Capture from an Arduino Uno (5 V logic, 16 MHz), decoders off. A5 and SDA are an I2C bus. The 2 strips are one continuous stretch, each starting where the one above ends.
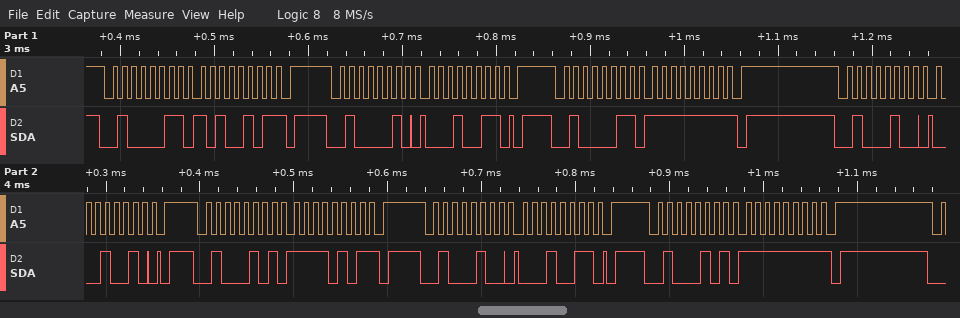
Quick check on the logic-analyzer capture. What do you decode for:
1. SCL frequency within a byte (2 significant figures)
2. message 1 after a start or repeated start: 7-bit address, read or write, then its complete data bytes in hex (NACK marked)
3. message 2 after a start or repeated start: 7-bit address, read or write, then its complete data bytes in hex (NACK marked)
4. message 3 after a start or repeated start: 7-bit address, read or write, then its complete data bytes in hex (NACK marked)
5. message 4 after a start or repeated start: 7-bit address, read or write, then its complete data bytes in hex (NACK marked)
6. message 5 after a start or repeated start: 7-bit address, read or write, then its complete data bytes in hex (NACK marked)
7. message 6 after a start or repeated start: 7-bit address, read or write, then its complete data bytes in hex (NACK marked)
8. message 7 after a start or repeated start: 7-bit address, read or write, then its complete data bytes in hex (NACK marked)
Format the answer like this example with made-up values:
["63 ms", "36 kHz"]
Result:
["100 kHz", "0x21 read: A5 NACK", "0x21 write: 13", "0x21 read: FF NACK", "0x22 write: 12", "0x22 read: F5 NACK", "0x22 write: 13", "0x22 read: FF NACK"]
